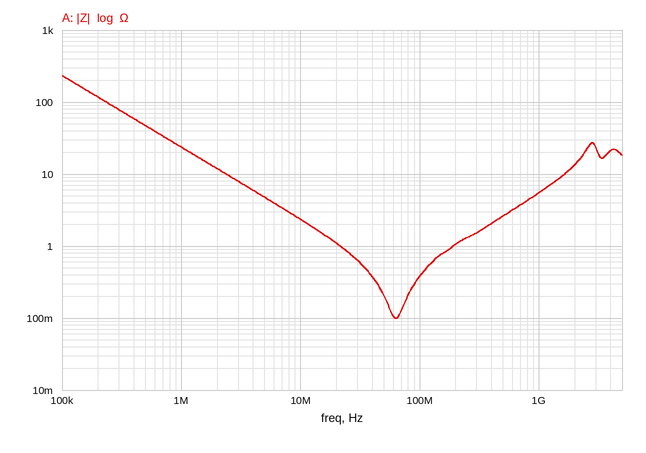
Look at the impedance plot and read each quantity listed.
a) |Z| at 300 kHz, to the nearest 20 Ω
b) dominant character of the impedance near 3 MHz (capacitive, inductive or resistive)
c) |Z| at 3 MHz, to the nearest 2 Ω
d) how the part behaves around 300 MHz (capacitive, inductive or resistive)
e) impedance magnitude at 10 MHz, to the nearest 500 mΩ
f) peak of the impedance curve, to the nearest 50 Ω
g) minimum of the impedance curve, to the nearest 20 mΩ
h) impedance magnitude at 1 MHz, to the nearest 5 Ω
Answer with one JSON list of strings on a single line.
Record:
["80 Ω", "capacitive", "8 Ω", "inductive", "2.5 Ω", "250 Ω", "100 mΩ", "25 Ω"]
